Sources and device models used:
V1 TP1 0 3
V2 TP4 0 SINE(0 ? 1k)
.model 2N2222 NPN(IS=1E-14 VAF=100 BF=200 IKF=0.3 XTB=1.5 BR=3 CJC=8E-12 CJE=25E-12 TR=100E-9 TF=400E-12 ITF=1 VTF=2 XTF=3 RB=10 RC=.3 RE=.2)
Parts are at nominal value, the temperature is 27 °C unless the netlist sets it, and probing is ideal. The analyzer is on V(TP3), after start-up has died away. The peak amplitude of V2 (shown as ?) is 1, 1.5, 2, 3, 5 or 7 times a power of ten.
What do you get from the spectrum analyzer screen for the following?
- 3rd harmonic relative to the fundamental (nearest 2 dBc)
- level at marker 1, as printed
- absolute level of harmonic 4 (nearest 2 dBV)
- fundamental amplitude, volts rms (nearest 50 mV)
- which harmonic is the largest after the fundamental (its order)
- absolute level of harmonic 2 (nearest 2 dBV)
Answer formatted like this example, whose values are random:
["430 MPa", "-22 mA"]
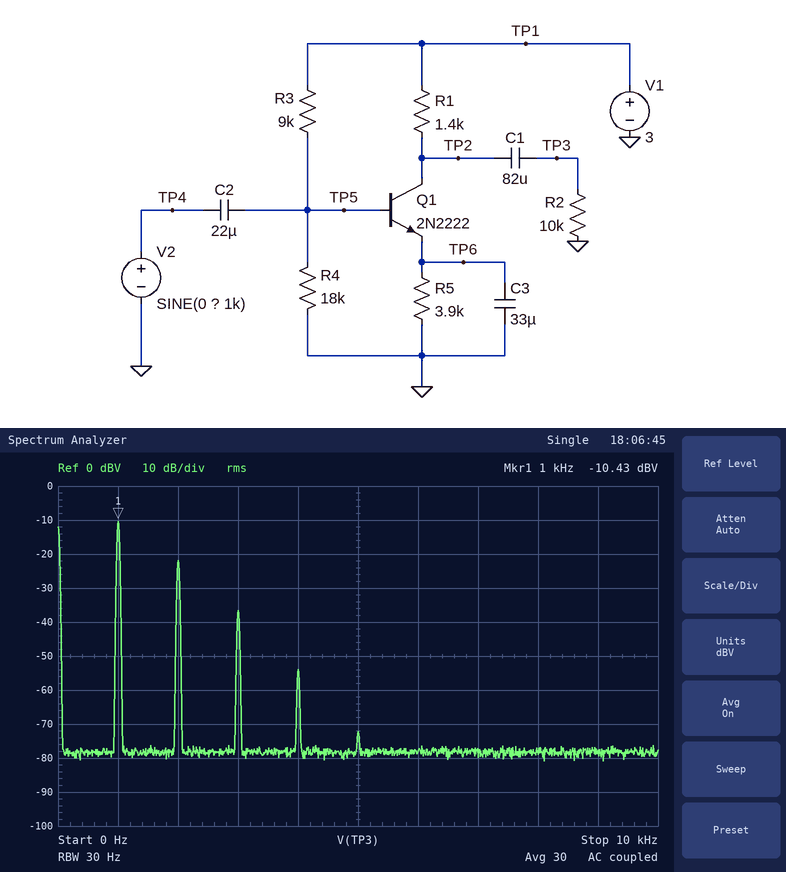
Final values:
["-26 dBc", "-10.43 dBV", "-54 dBV", "300 mV", "2", "-22 dBV"]
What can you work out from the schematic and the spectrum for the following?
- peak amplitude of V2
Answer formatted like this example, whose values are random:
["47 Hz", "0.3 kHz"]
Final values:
["30 mV"]
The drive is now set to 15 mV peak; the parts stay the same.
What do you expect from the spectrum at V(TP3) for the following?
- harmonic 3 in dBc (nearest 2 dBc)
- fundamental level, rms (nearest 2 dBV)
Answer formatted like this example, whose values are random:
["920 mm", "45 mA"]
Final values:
["-38 dBc", "-16 dBV"]
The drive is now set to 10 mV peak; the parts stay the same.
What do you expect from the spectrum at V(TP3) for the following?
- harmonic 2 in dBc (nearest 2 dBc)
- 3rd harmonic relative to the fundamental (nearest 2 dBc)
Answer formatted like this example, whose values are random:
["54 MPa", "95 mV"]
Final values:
["-20 dBc", "-44 dBc"]
